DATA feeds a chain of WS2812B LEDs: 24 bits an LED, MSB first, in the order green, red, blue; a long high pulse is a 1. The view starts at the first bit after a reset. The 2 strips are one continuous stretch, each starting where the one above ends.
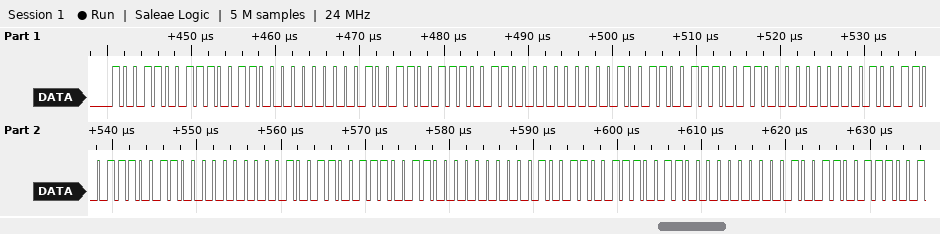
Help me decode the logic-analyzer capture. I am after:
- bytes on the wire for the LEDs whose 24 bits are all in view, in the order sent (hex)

99 CC 00 99 CC 00 99 CC 00 99 CC 00 99 CC 00 99 CC 00
